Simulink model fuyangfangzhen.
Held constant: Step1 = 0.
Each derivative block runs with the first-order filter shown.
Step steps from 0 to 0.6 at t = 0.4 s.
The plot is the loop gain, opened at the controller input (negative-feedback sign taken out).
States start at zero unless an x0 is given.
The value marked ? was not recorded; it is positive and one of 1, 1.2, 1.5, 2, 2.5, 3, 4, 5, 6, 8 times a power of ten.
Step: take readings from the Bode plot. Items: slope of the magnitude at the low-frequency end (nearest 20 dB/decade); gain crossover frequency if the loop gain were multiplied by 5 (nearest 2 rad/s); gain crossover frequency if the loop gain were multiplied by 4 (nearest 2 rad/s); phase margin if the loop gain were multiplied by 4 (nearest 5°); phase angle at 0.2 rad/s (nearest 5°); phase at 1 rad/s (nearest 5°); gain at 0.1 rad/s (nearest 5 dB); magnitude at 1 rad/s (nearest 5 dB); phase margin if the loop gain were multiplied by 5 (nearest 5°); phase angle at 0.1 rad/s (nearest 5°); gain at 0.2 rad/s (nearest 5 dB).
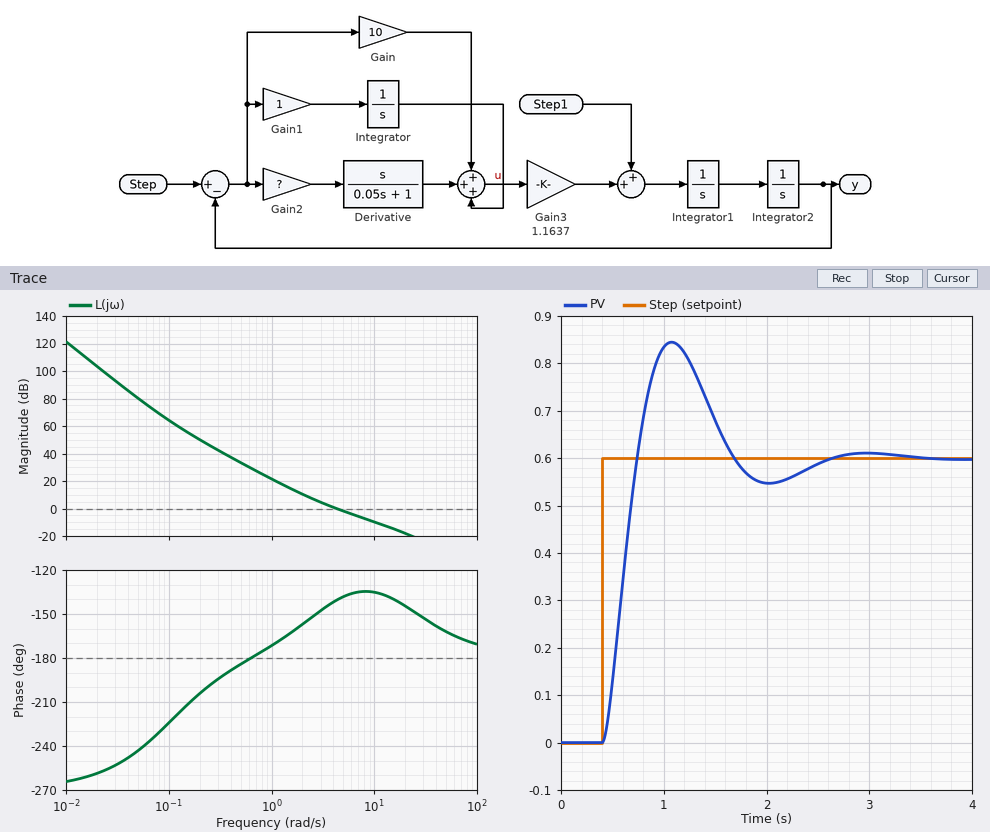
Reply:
-60 dB/decade
14 rad/s
12 rad/s
45°
-205°
-170°
65 dB
20 dB
40°
-225°
50 dB
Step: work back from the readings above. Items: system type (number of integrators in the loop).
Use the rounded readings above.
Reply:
3
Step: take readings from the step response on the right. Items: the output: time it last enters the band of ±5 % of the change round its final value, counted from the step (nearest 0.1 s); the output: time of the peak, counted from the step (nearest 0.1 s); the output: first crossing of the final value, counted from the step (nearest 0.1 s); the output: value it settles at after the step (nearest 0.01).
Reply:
1.9 s
0.7 s
0.3 s
0.60
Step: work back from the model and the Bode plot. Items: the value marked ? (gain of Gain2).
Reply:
2.5
